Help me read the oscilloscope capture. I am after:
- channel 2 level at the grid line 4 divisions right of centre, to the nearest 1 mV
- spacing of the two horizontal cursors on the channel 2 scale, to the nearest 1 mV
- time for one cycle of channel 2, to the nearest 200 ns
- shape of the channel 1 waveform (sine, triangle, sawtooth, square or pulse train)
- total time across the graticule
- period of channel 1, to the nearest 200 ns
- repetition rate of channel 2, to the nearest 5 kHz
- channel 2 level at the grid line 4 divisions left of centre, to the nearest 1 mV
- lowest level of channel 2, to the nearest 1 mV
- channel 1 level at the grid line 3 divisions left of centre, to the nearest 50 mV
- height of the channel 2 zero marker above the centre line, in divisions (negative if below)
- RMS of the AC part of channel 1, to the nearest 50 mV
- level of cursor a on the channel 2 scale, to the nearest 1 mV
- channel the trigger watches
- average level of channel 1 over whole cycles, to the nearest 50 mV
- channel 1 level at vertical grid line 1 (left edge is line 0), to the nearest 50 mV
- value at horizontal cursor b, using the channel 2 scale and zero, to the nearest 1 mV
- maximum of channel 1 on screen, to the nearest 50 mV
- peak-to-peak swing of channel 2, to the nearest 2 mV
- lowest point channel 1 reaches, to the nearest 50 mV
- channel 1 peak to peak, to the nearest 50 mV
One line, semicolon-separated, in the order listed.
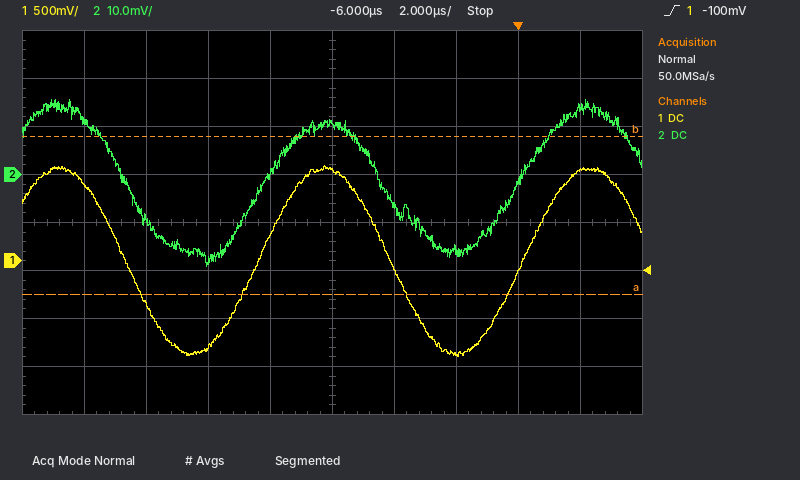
14 mV; 33 mV; 8.2 µs; sine; 20 µs; 8.6 µs; 120 kHz; 11 mV; -19 mV; -450 mV; +1.0 div; 700 mV; -25 mV; channel 1; 0 mV; 800 mV; 8 mV; 1.00 V; 34 mV; -1.00 V; 2.00 V
